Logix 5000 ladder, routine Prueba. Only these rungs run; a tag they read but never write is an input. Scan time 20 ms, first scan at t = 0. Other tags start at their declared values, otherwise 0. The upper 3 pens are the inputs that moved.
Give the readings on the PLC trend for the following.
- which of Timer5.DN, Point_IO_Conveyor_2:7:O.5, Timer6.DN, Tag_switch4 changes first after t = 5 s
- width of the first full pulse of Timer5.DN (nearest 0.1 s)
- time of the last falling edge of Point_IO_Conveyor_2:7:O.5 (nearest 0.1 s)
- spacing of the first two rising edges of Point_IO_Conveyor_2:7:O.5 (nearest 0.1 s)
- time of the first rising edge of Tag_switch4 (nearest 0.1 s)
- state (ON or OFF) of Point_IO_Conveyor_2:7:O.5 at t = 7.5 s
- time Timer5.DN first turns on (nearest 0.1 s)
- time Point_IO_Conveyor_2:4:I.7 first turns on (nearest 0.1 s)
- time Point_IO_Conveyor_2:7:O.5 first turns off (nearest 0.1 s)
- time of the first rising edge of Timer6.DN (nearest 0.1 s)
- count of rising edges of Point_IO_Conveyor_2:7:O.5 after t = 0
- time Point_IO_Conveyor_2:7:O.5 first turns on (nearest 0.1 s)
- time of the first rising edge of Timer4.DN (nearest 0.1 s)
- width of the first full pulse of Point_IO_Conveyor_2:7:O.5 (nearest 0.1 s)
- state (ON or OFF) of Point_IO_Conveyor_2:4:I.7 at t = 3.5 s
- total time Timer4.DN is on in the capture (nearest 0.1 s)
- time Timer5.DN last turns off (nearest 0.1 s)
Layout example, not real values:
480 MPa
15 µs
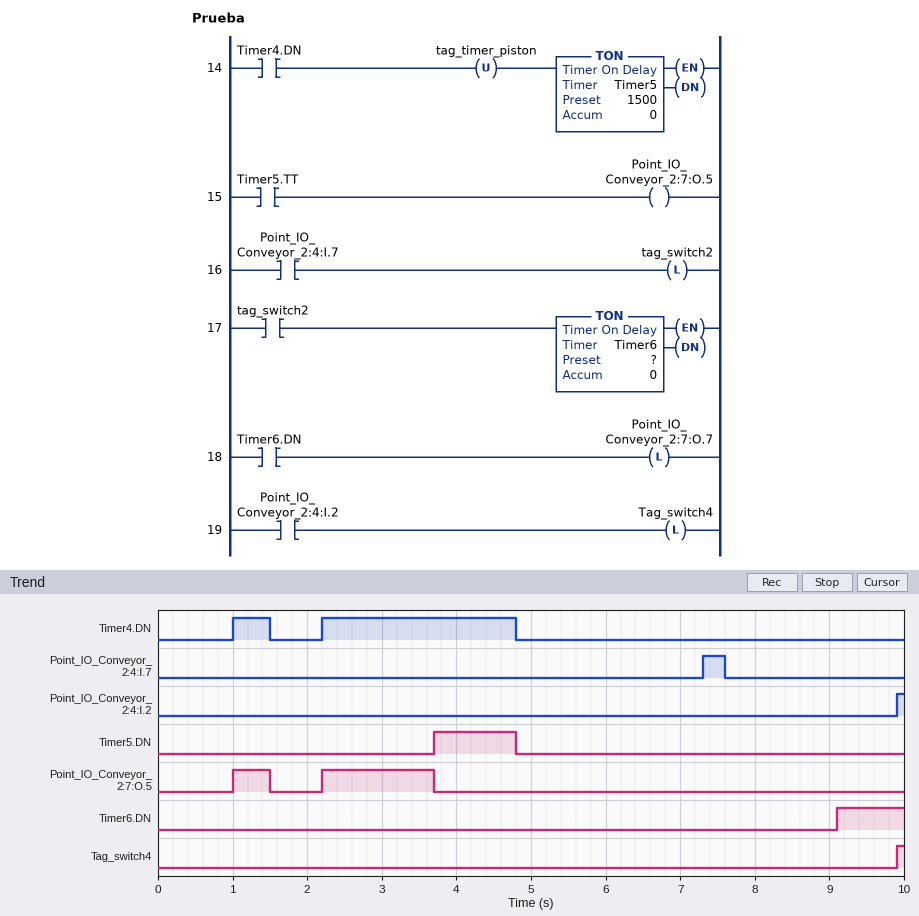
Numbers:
Timer6.DN
1.1 s
3.7 s
1.2 s
9.9 s
OFF
3.7 s
7.3 s
1.5 s
9.1 s
2
1.0 s
1.0 s
0.5 s
OFF
3.1 s
4.8 s
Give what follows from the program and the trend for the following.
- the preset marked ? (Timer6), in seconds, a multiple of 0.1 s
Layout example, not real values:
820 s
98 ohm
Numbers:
1.8 s
